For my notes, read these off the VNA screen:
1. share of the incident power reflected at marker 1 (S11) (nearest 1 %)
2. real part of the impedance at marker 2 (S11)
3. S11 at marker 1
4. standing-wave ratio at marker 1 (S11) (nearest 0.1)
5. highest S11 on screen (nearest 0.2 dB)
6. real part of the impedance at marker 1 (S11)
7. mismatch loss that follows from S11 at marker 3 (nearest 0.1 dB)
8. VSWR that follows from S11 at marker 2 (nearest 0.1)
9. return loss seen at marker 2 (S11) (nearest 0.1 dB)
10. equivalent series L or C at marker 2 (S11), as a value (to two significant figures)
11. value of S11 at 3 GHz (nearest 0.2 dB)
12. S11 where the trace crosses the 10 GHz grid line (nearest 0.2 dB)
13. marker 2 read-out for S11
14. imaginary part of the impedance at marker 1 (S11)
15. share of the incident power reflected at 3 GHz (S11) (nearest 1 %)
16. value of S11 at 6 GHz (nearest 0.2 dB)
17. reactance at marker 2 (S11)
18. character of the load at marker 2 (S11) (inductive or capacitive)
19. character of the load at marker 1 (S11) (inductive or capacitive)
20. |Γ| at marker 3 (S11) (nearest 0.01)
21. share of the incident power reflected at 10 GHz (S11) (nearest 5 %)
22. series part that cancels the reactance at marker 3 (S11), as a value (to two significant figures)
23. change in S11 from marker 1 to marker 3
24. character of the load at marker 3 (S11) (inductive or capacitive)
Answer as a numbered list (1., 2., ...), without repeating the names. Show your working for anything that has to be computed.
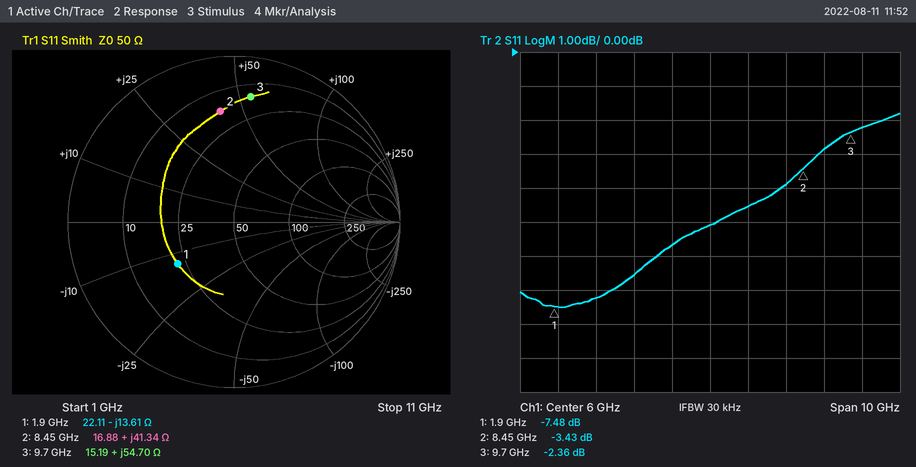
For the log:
1. 10^(-7.48/10) ≈ 18 %
2. 16.88 Ω
3. -7.48 dB
4. 2.5
5. -1.8 dB
6. 22.11 Ω
7. −10 log10(1 − 10^(-2.36/10)) ≈ 3.8 dB
8. (1 + 0.6738)/(1 − 0.6738) ≈ 5.1
9. 3.4 dB
10. L = 41.34 Ω/(2π × 8.45 GHz) ≈ 779 pH, so 780 pH to two significant figures
11. -7.2 dB
12. -2.2 dB
13. -3.43 dB
14. -13.61 Ω
15. 10^(-7.2/10) ≈ 19 %
16. -5.0 dB
17. +41.34 Ω
18. inductive
19. capacitive
20. 0.76
21. 10^(-2.2/10) ≈ 60 %
22. C = 1/(2π × 9.7 GHz × 54.7 Ω) ≈ 300 fF
23. -2.36 − (-7.48) = 5.12 dB
24. inductive
